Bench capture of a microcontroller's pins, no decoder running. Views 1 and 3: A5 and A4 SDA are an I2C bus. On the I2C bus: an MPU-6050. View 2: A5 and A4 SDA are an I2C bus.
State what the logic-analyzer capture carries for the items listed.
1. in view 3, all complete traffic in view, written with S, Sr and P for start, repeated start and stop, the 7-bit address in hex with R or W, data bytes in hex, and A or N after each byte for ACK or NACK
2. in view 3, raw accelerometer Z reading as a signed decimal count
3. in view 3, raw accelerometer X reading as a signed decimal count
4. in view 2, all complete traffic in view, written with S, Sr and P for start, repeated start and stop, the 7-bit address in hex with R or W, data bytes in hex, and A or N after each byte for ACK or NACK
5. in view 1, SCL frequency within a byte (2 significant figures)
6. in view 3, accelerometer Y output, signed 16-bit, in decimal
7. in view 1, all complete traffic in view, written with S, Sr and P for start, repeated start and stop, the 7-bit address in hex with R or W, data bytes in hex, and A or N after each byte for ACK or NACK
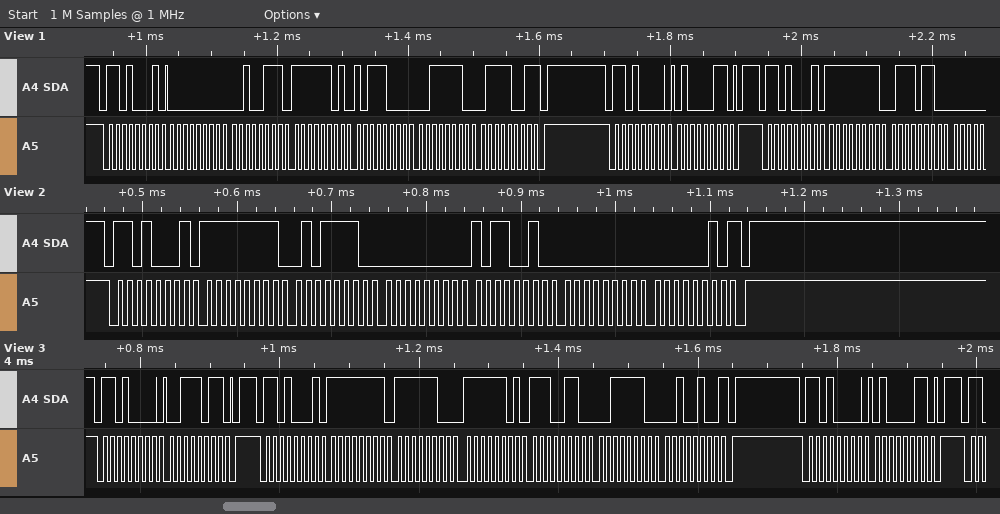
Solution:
S 68W A 3B A P S 68R A FF A FC A FD A E6 A 3E A 24 N P S 68W A 43 A P
15908
-4
S 68R A FF A 5E A 00 A B2 A 00 A 02 N P
100 kHz
-538
S 68R A 00 A 27 A FD A B8 A 3E A 79 N P S 68W A 43 A P S 68R A FF A 76 A
